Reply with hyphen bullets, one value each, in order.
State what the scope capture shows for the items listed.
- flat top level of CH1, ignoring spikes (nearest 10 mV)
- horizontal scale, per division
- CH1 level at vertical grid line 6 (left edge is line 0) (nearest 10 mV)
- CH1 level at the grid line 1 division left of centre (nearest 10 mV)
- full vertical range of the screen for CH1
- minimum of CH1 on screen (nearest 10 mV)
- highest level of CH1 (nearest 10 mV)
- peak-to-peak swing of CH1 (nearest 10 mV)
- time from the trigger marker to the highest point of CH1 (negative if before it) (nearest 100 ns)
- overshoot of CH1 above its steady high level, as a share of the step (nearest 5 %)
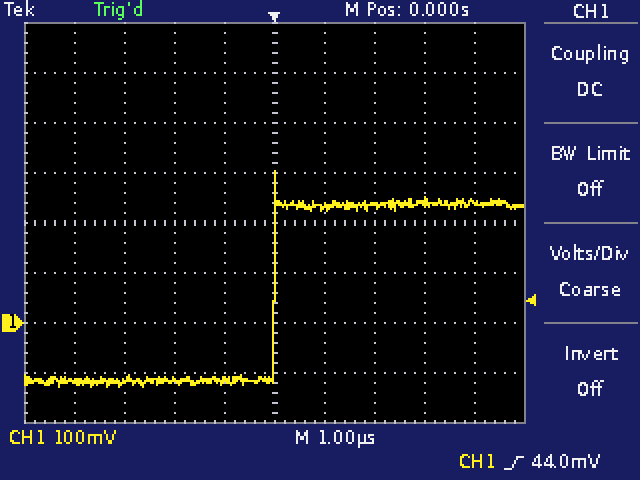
- 240 mV
- 1 µs
- 230 mV
- -120 mV
- 800 mV
- -130 mV
- 300 mV
- 430 mV
- 0.0 µs
- 20 %
